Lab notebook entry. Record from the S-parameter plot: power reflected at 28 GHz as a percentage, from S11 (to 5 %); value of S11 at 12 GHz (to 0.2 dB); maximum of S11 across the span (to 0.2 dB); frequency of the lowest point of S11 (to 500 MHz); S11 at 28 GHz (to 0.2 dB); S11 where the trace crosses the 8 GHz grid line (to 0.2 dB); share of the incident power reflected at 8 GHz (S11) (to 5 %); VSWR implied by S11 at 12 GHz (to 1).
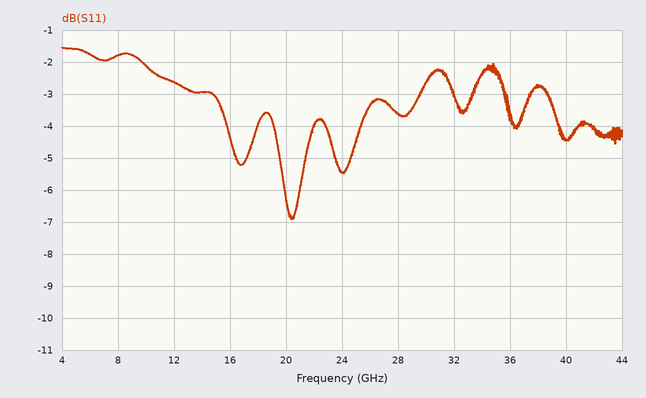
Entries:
45 %
-2.6 dB
-1.6 dB
20.5 GHz
-3.6 dB
-1.8 dB
65 %
7
